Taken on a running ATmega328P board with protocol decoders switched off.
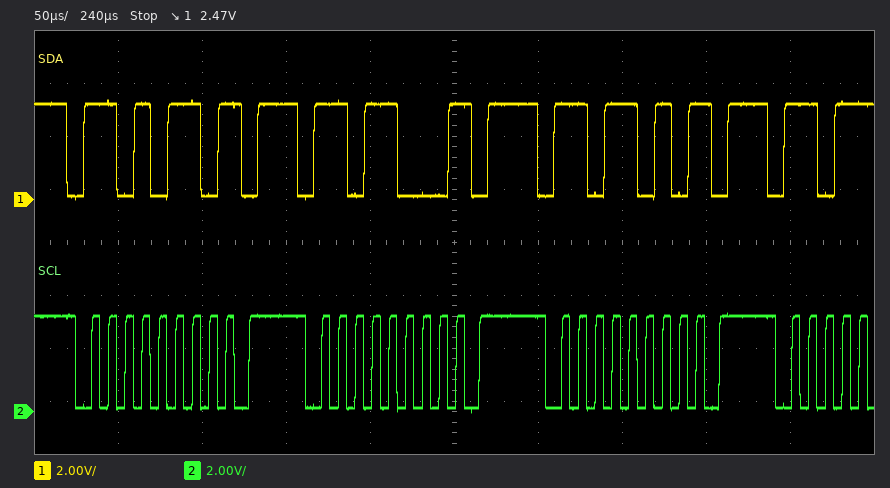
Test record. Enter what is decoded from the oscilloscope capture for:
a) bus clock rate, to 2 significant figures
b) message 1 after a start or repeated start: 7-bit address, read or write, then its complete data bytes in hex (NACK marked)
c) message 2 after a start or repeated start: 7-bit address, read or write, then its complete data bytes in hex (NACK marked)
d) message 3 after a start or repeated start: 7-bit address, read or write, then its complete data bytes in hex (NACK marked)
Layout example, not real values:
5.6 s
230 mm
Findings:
100 kHz
0x6B write NACK
0x6C write NACK
0x6D write NACK
